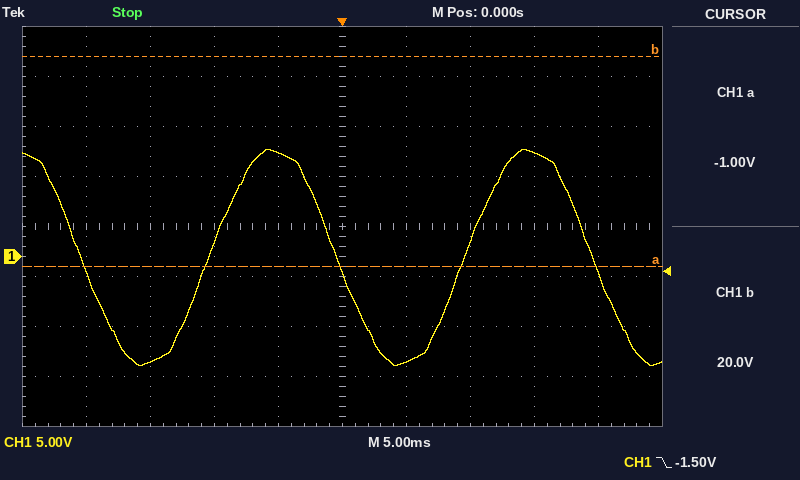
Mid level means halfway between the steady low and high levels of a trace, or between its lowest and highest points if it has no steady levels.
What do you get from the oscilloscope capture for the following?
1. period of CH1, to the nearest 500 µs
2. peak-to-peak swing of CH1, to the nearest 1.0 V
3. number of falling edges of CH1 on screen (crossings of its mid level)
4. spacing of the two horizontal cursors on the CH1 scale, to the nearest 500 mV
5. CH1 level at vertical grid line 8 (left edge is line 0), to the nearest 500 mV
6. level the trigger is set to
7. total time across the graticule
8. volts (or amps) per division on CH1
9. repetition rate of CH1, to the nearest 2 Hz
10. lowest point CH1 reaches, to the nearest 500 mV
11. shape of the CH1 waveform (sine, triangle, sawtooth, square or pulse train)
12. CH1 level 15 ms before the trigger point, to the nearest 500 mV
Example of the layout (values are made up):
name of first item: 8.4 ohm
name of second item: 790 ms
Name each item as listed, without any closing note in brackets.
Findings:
period of CH1, to the nearest 500 µs: 20.0 ms
peak-to-peak swing of CH1, to the nearest 1.0 V: 22.0 V
number of falling edges of CH1 on screen: 3
spacing of the two horizontal cursors on the CH1 scale, to the nearest 500 mV: 21.0 V
CH1 level at vertical grid line 8 (left edge is line 0), to the nearest 500 mV: 10.5 V
level the trigger is set to: -1.50 V
total time across the graticule: 50 ms
volts (or amps) per division on CH1: 5 V
repetition rate of CH1, to the nearest 2 Hz: 50 Hz
lowest point CH1 reaches, to the nearest 500 mV: -11.0 V
shape of the CH1 waveform: sine
CH1 level 15 ms before the trigger point, to the nearest 500 mV: -10.5 V
